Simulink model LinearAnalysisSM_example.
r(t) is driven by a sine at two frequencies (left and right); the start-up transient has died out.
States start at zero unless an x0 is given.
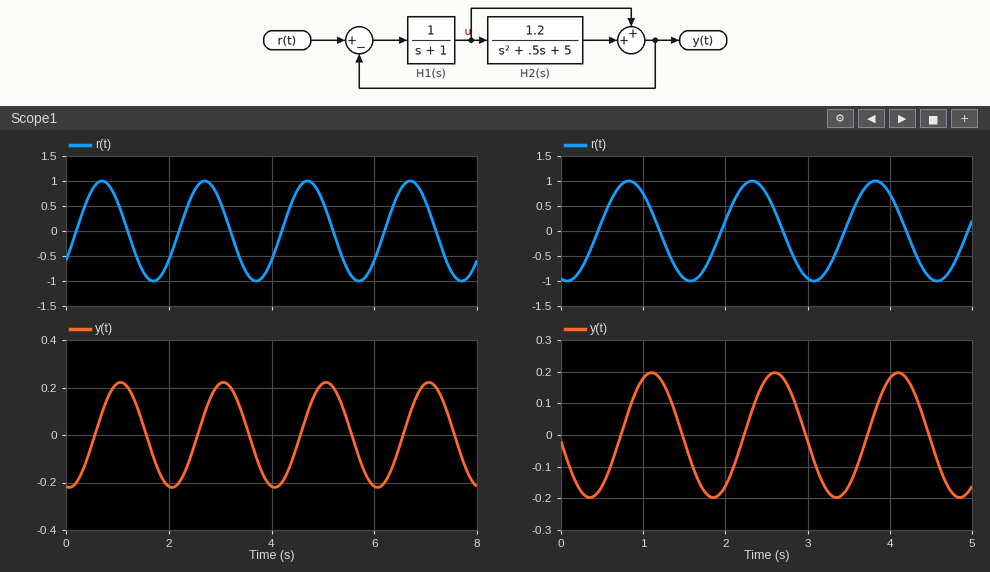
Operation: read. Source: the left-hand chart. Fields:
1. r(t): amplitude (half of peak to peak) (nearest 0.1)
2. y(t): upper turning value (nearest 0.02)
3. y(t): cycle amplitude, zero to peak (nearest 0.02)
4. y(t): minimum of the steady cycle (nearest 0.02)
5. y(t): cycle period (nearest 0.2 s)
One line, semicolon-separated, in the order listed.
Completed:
1.0; 0.22; 0.22; -0.22; 2.0 s
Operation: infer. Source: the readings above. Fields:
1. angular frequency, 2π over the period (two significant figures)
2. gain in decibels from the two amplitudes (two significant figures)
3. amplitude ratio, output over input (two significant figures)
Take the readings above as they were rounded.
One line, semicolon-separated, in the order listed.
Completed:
3.1 rad/s; -13 dB; 0.22
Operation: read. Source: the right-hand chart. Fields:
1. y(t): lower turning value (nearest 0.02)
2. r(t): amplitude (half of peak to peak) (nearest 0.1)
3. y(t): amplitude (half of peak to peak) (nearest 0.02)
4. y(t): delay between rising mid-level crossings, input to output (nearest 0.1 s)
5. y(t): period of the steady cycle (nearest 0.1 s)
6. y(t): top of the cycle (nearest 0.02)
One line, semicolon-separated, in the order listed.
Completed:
-0.20; 1.0; 0.20; 0.3 s; 1.5 s; 0.20
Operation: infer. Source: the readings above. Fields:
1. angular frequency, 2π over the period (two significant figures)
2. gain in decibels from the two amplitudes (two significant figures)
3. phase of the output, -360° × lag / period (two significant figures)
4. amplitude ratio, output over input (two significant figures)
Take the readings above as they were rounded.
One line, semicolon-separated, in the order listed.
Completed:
4.2 rad/s; -14 dB; -72°; 0.20
